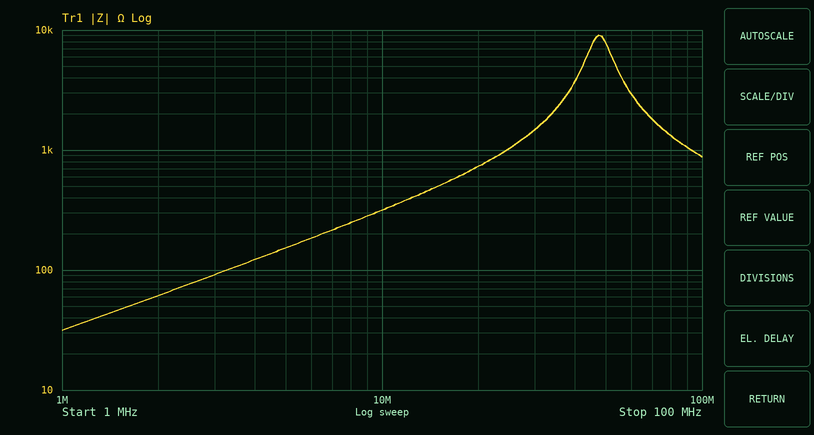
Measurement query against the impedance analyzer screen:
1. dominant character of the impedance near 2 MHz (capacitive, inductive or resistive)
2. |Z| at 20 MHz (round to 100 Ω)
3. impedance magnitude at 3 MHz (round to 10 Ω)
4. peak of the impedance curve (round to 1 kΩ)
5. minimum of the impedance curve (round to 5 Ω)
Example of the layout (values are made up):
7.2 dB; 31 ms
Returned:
inductive; 700 Ω; 90 Ω; 9 kΩ; 30 Ω
